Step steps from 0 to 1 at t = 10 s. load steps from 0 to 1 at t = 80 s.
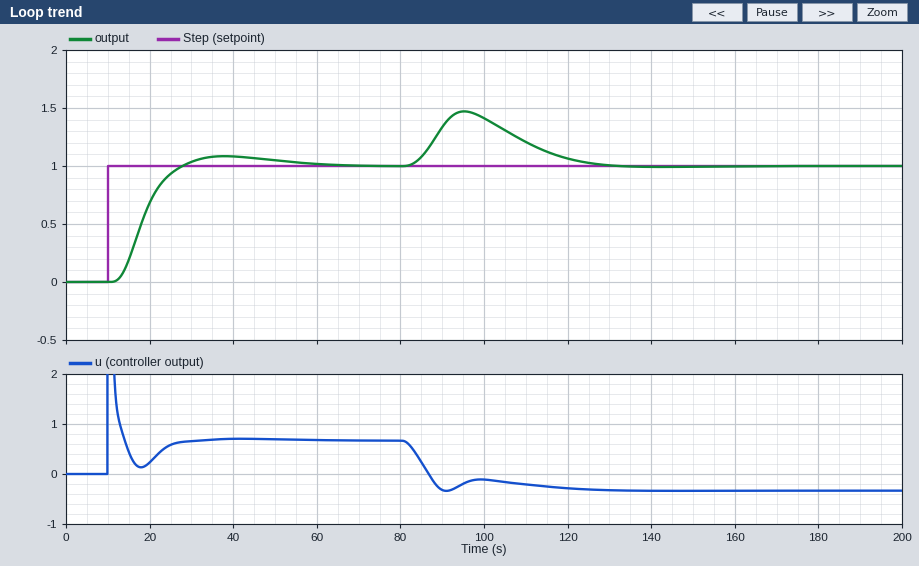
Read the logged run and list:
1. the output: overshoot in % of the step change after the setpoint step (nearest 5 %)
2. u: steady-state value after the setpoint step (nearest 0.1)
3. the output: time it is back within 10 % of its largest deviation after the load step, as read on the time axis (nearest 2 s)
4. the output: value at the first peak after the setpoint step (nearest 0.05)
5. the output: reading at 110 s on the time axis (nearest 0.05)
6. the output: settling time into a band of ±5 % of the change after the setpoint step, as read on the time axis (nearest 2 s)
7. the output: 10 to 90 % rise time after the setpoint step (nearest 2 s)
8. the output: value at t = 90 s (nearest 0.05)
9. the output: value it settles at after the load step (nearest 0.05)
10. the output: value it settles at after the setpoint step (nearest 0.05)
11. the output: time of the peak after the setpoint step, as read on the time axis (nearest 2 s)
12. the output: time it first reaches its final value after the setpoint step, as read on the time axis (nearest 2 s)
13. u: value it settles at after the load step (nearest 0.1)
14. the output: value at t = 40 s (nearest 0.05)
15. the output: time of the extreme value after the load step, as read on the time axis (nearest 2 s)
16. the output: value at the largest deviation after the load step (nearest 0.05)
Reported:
10 %
0.7
122 s
1.10
1.20
50 s
10 s
1.35
1.00
1.00
38 s
28 s
-0.3
1.10
96 s
1.45
